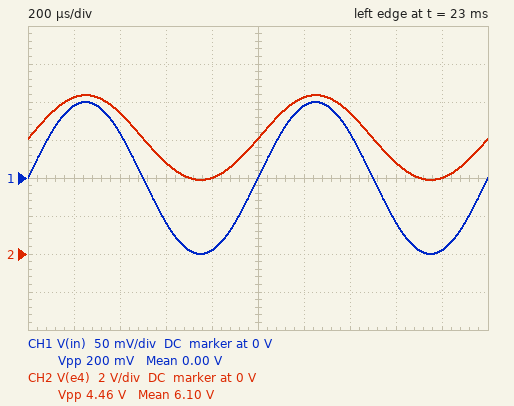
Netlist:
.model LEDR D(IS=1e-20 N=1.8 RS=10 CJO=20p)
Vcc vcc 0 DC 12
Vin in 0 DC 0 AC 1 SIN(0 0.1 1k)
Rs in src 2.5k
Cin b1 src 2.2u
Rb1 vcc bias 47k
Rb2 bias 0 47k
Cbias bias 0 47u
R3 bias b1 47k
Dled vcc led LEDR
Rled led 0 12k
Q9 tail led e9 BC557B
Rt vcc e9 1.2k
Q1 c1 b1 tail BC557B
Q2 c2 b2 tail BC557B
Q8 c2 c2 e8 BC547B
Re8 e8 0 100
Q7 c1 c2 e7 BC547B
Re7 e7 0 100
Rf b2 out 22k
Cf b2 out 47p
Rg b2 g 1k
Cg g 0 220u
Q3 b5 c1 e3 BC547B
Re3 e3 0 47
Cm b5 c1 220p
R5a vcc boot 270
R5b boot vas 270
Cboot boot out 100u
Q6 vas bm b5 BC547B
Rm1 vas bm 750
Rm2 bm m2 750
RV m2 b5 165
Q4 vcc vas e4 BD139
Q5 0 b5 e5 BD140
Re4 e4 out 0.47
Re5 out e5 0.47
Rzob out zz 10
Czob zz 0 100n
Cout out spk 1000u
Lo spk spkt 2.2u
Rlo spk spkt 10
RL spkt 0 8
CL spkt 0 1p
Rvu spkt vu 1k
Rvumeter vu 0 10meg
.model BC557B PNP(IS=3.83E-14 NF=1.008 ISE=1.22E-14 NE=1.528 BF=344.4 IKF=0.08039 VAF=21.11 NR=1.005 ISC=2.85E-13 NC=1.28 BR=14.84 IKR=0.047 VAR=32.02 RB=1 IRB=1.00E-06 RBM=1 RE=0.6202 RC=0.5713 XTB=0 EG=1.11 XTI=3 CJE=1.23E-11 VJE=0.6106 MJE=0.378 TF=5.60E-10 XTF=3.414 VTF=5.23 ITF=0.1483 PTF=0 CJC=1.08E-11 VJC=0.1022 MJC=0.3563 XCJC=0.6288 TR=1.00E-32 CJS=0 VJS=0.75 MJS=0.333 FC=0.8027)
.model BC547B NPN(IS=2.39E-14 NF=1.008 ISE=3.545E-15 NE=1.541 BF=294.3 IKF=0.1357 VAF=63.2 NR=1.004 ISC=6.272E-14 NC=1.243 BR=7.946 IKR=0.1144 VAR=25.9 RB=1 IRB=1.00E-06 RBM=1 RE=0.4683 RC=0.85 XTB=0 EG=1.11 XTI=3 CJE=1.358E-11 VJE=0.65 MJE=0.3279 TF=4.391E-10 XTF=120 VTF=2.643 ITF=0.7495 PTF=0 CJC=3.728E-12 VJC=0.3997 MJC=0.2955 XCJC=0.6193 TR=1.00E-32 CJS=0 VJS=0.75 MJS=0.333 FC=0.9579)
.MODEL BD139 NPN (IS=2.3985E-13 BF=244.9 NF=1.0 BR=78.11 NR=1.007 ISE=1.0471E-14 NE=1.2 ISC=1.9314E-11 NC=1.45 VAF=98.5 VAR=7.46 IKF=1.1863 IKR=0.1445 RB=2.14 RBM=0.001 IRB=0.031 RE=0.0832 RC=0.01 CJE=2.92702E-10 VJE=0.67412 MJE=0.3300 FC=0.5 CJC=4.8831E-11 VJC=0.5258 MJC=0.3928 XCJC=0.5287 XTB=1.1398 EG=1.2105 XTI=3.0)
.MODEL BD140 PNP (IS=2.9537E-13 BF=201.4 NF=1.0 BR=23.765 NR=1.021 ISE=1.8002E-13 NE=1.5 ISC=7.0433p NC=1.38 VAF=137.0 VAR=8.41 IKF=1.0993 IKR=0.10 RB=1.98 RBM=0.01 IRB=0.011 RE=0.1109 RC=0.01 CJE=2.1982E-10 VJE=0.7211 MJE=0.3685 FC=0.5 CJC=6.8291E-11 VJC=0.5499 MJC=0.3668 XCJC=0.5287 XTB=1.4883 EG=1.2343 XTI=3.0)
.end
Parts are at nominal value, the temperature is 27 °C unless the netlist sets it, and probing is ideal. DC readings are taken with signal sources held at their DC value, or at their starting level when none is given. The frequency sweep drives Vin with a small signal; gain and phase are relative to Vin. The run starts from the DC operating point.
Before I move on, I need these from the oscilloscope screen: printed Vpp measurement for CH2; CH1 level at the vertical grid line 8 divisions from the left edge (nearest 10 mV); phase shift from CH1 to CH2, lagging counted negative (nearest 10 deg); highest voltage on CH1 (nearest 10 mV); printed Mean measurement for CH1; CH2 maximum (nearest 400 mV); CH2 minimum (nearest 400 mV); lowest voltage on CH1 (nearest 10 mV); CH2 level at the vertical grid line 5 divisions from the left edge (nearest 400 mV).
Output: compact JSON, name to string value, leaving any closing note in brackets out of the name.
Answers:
{"printed Vpp measurement for CH2": "4.46 V", "CH1 level at the vertical grid line 8 divisions from the left edge": "-60 mV", "phase shift from CH1 to CH2, lagging counted negative": "0 deg", "highest voltage on CH1": "100 mV", "printed Mean measurement for CH1": "0.00 V", "CH2 maximum": "8.4 V", "CH2 minimum": "4.0 V", "lowest voltage on CH1": "-100 mV", "CH2 level at the vertical grid line 5 divisions from the left edge": "6.0 V"}
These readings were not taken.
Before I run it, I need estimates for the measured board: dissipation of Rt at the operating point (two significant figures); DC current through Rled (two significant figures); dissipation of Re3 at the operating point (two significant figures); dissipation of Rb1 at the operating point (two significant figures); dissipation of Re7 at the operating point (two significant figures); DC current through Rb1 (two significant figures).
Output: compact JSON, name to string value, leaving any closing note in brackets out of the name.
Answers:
{"dissipation of Rt at the operating point": "1.2 mW", "DC current through Rled": "850 µA", "dissipation of Re3 at the operating point": "4.5 mW", "dissipation of Rb1 at the operating point": "760 µW", "dissipation of Re7 at the operating point": "23 µW", "DC current through Rb1": "130 µA"}
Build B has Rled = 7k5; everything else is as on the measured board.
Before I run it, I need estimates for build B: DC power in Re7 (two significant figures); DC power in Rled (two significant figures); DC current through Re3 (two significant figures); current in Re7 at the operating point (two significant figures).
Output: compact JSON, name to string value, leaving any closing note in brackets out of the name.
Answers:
{"DC power in Re7": "24 µW", "DC power in Rled": "14 mW", "DC current through Re3": "9.8 mA", "current in Re7 at the operating point": "490 µA"}
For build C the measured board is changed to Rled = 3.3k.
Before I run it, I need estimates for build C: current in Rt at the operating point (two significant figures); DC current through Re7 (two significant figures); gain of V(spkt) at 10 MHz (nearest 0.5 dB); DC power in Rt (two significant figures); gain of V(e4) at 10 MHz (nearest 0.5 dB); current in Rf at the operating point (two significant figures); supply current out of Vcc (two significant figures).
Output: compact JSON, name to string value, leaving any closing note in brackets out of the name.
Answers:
{"current in Rt at the operating point": "1.1 mA", "DC current through Re7": "510 µA", "gain of V(spkt) at 10 MHz": "-17.0 dB", "DC power in Rt": "1.4 mW", "gain of V(e4) at 10 MHz": "-9.5 dB", "current in Rf at the operating point": "1.3 µA", "supply current out of Vcc": "29 mA"}
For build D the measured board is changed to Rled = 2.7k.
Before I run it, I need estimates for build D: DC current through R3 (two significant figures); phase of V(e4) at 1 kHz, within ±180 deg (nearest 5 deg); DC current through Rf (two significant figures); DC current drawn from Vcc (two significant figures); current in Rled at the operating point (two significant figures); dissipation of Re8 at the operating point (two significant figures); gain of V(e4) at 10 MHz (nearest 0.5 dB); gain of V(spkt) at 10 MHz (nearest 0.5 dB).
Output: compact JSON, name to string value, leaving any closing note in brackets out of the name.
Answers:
{"DC current through R3": "1.4 µA", "phase of V(e4) at 1 kHz, within ±180 deg": "0 deg", "DC current through Rf": "1.3 µA", "DC current drawn from Vcc": "30 mA", "current in Rled at the operating point": "3.7 mA", "dissipation of Re8 at the operating point": "27 µW", "gain of V(e4) at 10 MHz": "-9.5 dB", "gain of V(spkt) at 10 MHz": "-17.0 dB"}
